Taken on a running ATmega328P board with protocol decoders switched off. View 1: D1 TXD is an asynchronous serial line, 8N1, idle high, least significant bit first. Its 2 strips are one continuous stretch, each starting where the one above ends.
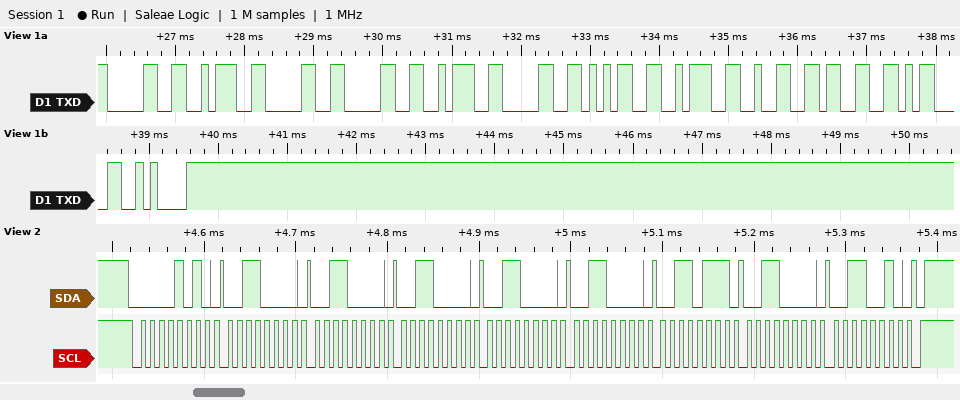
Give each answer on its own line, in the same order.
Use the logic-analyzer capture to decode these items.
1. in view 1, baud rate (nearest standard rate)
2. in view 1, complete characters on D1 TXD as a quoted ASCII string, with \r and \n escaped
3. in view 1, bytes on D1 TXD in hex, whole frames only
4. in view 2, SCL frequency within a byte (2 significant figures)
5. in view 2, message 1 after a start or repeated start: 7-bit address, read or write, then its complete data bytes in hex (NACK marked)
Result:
9600 baud
"0:00:05:23\r\n"
0x30 0x3A 0x30 0x30 0x3A 0x30 0x35 0x3A 0x32 0x33 0x0D 0x0A
100 kHz
0x05 write: 30 30 30 30 30 37 30 32
